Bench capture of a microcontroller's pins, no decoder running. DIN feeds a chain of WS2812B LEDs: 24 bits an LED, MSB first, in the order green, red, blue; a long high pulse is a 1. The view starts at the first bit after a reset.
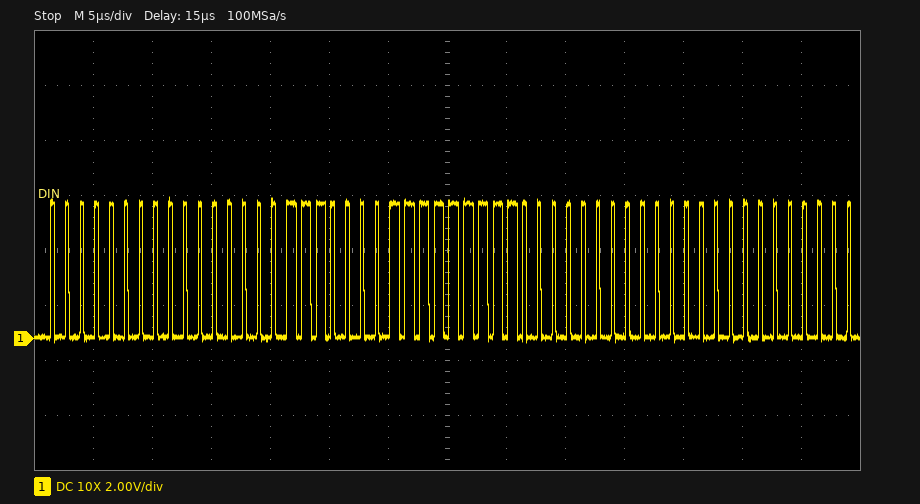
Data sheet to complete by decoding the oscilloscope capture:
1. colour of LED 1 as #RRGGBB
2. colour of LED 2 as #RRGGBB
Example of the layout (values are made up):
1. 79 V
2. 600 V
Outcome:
1. #0000E1
2. #00FF00
